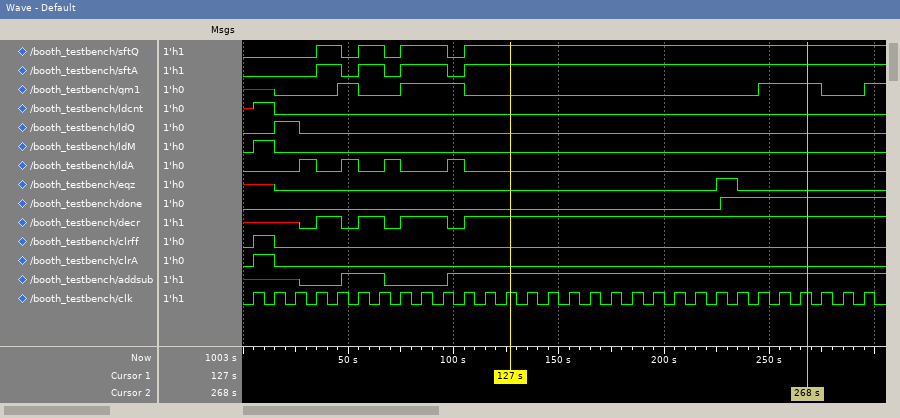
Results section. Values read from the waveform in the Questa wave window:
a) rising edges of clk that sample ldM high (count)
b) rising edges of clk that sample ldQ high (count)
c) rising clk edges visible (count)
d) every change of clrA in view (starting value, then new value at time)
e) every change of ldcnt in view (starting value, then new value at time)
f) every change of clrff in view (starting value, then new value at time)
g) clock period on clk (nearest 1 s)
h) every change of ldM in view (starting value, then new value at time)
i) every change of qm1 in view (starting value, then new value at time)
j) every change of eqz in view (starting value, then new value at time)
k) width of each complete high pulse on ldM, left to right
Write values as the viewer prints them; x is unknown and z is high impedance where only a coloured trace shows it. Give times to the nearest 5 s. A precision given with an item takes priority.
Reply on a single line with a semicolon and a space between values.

1; 1; 30; 0, 1 at 5 s, 0 at 15 s; x, 1 at 5 s, 0 at 15 s; 0, 1 at 5 s, 0 at 15 s; 10 s; 0, 1 at 5 s, 0 at 15 s; x, 0 at 15 s, 1 at 45 s, 0 at 55 s, 1 at 75 s, 0 at 105 s, 1 at 245 s, 0 at 275 s, 1 at 295 s; x, 0 at 15 s, 1 at 225 s, 0 at 235 s; 10 s
